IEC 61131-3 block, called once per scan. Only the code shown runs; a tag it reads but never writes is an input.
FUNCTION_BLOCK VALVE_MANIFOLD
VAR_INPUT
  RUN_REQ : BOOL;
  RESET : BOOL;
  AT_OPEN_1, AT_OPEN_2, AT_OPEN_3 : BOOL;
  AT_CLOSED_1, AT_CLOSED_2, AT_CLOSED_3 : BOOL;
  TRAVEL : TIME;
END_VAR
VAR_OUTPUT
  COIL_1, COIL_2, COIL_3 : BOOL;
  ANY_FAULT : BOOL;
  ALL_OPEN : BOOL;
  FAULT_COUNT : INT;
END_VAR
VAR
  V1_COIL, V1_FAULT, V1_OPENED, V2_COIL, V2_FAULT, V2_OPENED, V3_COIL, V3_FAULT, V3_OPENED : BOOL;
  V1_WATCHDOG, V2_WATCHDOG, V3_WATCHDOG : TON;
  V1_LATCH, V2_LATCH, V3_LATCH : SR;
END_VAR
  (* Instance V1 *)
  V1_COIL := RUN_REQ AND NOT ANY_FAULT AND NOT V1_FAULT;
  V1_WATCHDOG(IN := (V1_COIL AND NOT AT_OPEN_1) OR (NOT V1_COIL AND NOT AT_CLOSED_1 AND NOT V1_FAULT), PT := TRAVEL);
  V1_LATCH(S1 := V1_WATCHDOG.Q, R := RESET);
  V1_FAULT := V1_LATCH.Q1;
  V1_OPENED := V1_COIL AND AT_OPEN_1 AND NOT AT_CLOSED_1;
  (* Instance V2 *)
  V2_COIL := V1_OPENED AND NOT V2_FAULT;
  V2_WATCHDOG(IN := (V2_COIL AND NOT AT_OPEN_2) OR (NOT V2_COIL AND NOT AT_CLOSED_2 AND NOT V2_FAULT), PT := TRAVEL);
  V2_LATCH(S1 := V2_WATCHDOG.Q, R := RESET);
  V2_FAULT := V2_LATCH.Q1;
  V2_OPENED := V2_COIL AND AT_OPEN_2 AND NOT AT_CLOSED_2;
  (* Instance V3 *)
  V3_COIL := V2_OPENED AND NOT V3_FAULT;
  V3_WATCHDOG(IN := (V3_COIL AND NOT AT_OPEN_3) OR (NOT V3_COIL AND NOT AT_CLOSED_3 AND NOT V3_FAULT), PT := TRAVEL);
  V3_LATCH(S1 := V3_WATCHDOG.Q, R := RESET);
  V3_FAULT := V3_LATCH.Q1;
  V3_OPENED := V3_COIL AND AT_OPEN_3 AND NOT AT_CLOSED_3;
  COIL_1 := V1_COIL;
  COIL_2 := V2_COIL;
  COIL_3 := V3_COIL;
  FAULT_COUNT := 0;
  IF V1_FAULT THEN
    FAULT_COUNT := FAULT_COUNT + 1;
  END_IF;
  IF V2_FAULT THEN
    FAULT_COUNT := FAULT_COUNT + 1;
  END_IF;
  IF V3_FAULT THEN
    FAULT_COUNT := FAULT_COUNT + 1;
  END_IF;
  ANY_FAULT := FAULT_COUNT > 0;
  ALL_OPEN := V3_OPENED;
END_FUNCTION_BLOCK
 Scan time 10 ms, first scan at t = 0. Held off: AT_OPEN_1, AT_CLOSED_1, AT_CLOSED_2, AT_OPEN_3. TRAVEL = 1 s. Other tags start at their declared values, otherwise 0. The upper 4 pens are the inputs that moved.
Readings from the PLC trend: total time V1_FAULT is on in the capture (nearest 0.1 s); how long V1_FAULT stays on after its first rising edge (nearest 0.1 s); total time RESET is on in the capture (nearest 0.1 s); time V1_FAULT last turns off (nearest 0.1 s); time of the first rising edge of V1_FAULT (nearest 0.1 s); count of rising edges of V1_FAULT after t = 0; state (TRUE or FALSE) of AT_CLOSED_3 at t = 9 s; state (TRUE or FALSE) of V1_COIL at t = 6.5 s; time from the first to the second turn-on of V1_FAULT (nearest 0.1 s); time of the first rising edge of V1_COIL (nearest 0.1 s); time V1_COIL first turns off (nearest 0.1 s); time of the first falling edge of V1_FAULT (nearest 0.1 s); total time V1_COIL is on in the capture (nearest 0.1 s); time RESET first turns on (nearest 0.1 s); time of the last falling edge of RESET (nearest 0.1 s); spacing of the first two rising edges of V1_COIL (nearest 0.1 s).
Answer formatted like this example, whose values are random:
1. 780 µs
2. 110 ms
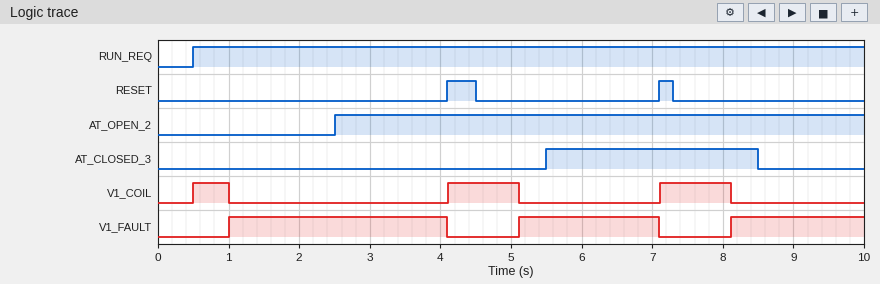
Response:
1. 7.0 s
2. 3.1 s
3. 0.6 s
4. 7.1 s
5. 1.0 s
6. 3
7. FALSE
8. FALSE
9. 4.1 s
10. 0.5 s
11. 1.0 s
12. 4.1 s
13. 2.5 s
14. 4.1 s
15. 7.3 s
16. 3.6 s
